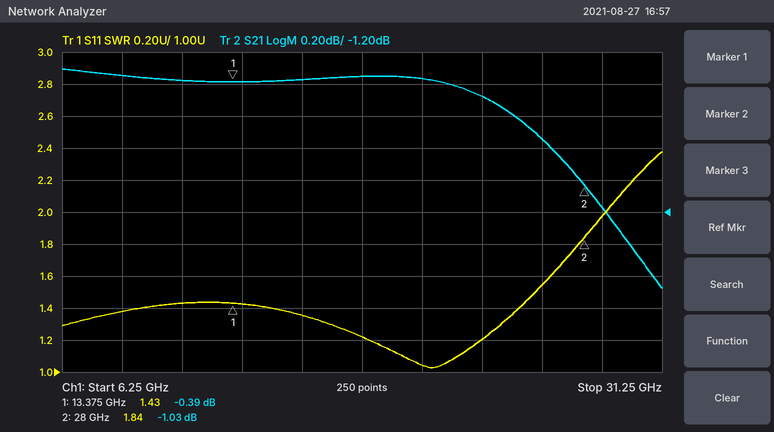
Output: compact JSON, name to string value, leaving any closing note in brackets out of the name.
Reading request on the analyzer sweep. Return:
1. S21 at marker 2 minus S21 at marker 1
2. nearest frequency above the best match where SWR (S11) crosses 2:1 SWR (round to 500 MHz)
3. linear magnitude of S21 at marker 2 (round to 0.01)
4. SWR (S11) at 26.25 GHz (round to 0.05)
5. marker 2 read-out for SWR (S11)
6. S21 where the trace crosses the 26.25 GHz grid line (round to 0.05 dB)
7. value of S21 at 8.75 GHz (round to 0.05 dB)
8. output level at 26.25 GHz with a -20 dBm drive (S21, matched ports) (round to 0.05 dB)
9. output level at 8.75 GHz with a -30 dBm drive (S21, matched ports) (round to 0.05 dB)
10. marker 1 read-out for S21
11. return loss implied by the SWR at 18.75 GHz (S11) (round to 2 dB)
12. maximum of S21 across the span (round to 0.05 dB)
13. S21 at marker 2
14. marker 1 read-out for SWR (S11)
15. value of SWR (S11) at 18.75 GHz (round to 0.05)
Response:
{"S21 at marker 2 minus S21 at marker 1": "-0.64 dB", "nearest frequency above the best match where SWR (S11) crosses 2:1 SWR": "29.0 GHz", "linear magnitude of S21 at marker 2": "0.89", "SWR (S11) at 26.25 GHz": "1.55", "marker 2 read-out for SWR": "1.84", "S21 where the trace crosses the 26.25 GHz grid line": "-0.75 dB", "value of S21 at 8.75 GHz": "-0.35 dB", "output level at 26.25 GHz with a -20 dBm drive (S21, matched ports)": "-20.75 dBm", "output level at 8.75 GHz with a -30 dBm drive (S21, matched ports)": "-30.35 dBm", "marker 1 read-out for S21": "-0.39 dB", "return loss implied by the SWR at 18.75 GHz (S11)": "20 dB", "maximum of S21 across the span": "-0.30 dB", "S21 at marker 2": "-1.03 dB", "marker 1 read-out for SWR": "1.43", "value of SWR (S11) at 18.75 GHz": "1.20"}
